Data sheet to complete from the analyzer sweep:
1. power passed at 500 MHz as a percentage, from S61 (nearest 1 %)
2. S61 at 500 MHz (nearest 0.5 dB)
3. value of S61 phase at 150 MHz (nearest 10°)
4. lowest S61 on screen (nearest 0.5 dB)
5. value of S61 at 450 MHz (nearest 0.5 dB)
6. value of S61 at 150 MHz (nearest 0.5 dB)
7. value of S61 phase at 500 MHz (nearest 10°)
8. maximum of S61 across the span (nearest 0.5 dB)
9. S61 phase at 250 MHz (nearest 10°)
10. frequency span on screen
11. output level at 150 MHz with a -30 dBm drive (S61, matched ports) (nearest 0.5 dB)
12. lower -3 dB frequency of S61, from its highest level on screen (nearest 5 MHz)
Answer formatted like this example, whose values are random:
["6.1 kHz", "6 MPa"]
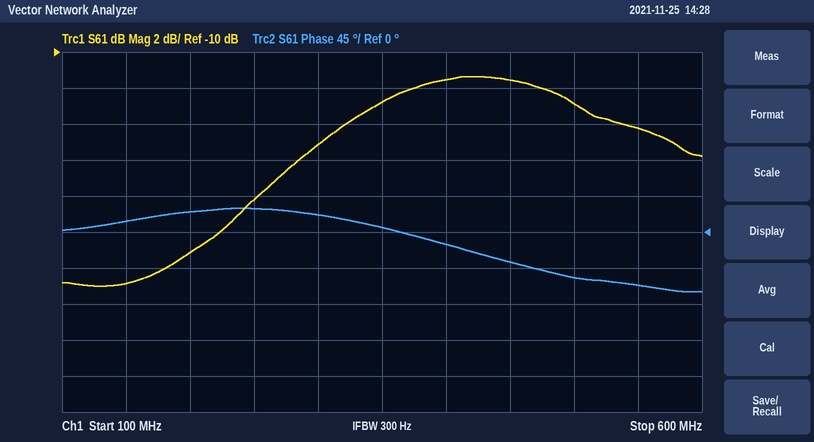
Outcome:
["5 %", "-13.0 dB", "10°", "-23.0 dB", "-11.5 dB", "-23.0 dB", "-60°", "-11.5 dB", "30°", "500 MHz", "-53.0 dBm", "315 MHz"]
